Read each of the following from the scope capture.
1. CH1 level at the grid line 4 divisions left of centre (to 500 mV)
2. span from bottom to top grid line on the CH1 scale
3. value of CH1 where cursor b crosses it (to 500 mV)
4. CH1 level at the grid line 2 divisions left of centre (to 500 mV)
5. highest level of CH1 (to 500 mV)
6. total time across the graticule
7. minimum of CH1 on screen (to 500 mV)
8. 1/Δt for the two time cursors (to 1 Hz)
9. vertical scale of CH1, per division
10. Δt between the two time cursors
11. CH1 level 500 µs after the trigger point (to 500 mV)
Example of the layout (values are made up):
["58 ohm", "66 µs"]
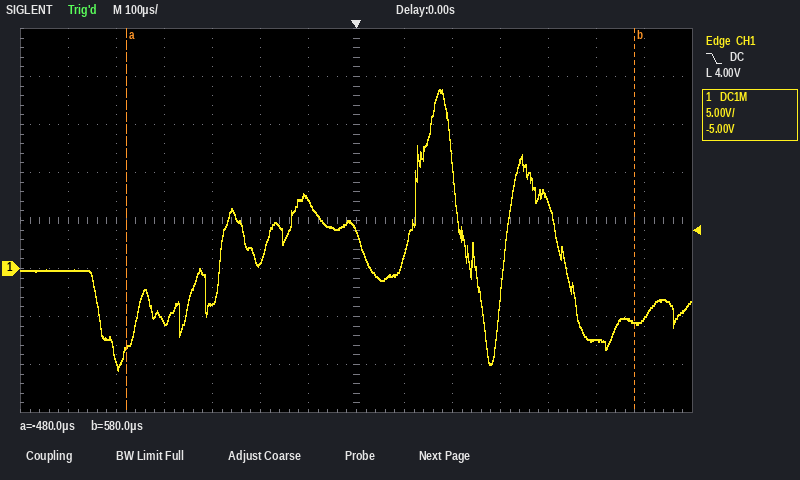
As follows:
["-5.5 V", "40 V", "-5.5 V", "500 mV", "18.5 V", "1.4 ms", "-10.5 V", "943 Hz", "5 V", "1.06 ms", "-7.5 V"]
